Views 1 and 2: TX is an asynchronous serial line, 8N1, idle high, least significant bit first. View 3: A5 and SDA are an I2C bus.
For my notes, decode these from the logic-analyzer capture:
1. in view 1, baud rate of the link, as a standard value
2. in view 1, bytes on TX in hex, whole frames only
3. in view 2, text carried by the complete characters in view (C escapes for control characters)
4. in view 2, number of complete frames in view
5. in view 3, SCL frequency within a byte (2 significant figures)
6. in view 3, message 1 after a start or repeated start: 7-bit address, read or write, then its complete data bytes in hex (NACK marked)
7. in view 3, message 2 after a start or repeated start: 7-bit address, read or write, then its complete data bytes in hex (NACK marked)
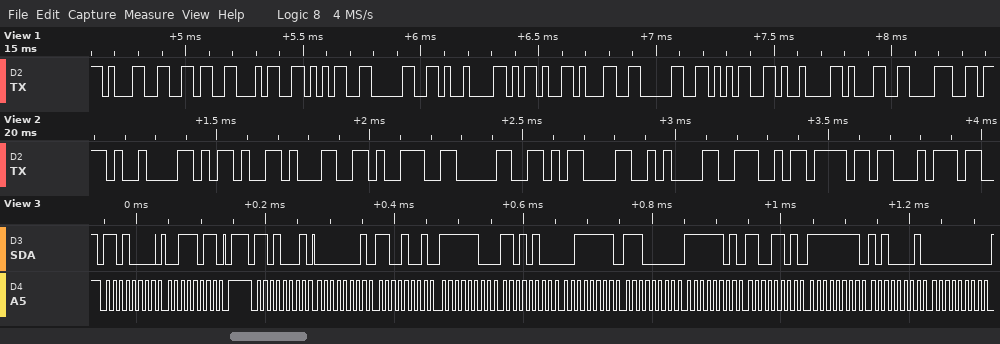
38400 baud
31 36 34 35 30 09 2D 31 30 35 09 31 38
"\t-190\r\nNot"
10
100 kHz
0x68 write: 3B
0x68 read: 01 C9 FC D4 3F E0 FD CD FF A1 00
